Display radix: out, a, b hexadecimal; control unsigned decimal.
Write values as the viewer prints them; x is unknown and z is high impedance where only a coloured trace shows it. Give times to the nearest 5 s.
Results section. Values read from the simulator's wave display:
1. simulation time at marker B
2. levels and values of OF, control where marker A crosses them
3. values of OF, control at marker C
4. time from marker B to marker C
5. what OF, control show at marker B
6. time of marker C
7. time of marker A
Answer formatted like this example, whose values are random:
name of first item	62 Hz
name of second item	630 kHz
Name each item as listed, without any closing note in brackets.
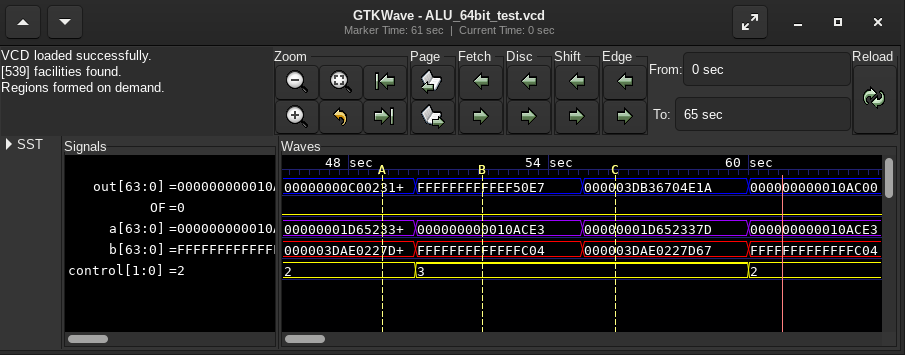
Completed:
simulation time at marker B	50 s
levels and values of OF, control where marker A crosses them	OF=0, control=2
values of OF, control at marker C	OF=0, control=3
time from marker B to marker C	5 s
what OF, control show at marker B	OF=0, control=3
time of marker C	55 s
time of marker A	50 s
